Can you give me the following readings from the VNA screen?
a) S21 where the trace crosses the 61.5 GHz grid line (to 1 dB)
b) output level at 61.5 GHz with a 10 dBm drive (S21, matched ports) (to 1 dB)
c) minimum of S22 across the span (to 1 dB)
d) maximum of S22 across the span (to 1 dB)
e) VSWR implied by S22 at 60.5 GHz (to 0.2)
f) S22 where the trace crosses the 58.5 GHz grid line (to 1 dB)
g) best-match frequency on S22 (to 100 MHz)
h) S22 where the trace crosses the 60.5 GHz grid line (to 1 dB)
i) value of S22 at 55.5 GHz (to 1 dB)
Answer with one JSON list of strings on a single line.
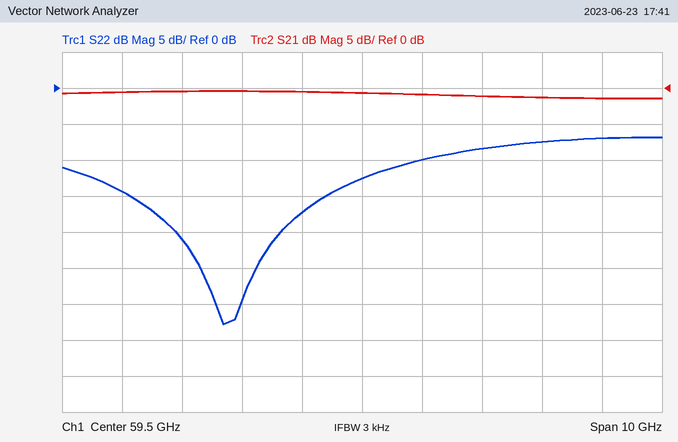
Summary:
["-1 dB", "9 dBm", "-33 dB", "-7 dB", "2.0", "-17 dB", "57.2 GHz", "-10 dB", "-14 dB"]
